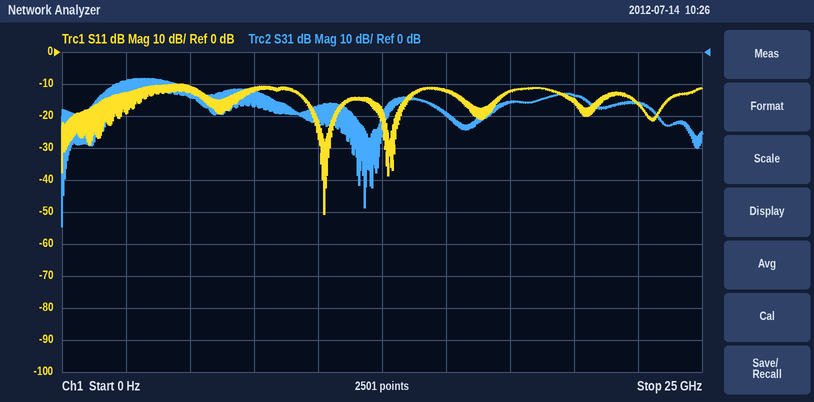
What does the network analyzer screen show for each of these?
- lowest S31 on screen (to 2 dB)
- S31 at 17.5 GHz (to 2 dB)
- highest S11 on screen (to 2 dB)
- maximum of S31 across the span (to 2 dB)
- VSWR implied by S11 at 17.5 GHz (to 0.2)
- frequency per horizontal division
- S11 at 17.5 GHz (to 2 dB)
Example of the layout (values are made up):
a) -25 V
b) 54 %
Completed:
a) -54 dB
b) -16 dB
c) -10 dB
d) -8 dB
e) 1.6
f) 2.5 GHz
g) -12 dB
